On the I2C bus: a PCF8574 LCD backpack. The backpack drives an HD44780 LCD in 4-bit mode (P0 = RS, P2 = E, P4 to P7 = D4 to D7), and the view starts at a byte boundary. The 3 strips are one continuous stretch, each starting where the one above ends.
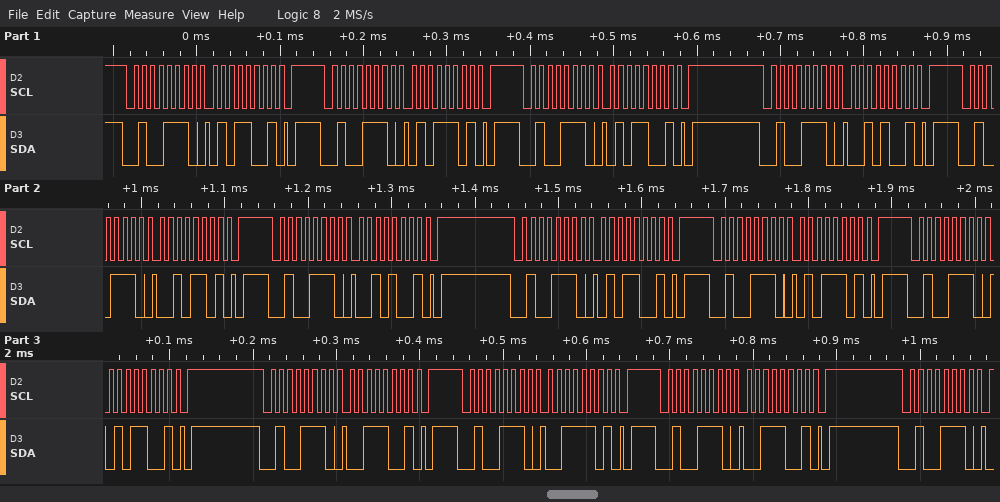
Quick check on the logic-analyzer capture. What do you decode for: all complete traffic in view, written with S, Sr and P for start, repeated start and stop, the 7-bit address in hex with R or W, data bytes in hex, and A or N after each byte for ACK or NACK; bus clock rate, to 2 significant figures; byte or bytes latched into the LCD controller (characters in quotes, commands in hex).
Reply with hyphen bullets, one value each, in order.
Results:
- S 27W A 59 A P S 27W A 5D A P S 27W A 59 A P S 27W A 29 A P S 27W A 2D A P S 27W A 29 A P S 27W A 59 A P S 27W A 5D A P S 27W A 59 A P S 27W A 39 A P S 27W A 3D A P S 27W A 39 A P S 27W A
- 100 kHz
- 'R' 'S'
